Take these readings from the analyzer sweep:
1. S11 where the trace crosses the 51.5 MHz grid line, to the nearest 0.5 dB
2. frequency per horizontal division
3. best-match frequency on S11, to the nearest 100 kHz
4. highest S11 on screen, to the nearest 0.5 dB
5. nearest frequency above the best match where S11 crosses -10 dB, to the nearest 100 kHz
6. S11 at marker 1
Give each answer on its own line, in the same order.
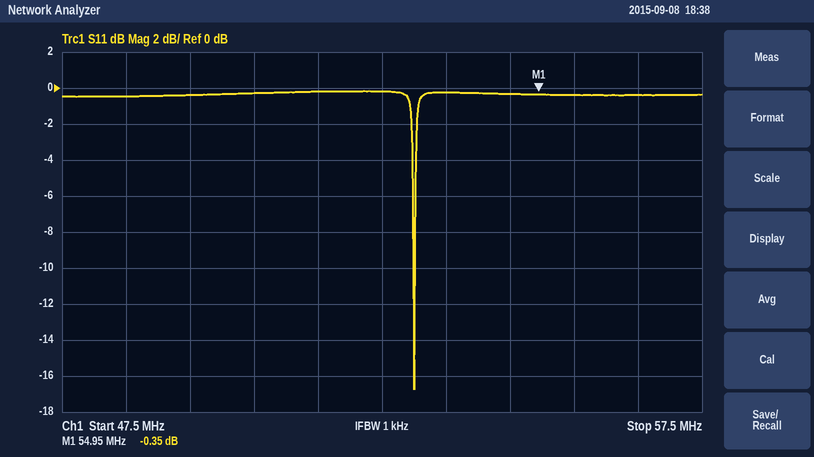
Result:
0.0 dB
1 MHz
53.0 MHz
0.0 dB
53.0 MHz
-0.35 dB
